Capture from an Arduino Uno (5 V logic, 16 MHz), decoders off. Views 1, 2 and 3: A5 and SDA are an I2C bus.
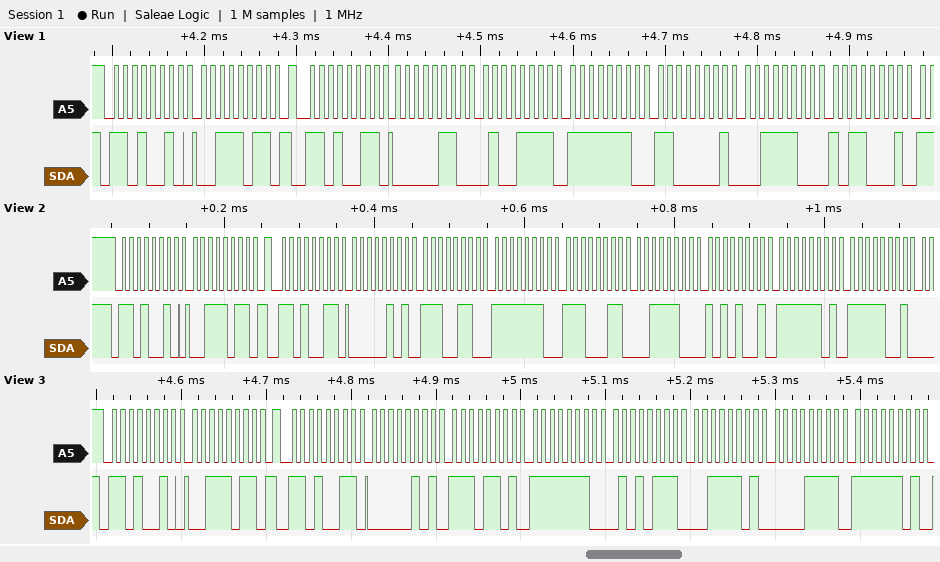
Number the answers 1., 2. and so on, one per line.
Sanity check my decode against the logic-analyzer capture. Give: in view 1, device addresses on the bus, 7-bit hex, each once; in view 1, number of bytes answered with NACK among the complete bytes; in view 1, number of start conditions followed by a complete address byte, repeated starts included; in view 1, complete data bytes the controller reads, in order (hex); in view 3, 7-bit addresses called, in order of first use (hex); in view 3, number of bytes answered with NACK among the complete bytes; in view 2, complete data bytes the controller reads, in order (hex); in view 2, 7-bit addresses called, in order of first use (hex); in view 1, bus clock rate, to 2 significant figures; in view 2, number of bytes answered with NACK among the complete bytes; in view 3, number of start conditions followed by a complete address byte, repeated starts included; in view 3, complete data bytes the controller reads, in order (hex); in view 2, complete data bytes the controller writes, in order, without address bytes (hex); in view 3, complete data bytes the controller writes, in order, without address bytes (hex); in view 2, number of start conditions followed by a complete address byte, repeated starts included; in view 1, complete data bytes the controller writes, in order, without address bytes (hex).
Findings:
1. 0x69
2. 0
3. 2
4. 06 4F FE C1 3C B1
5. 0x69
6. 0
7. 05 E6 FE E3 3C A9 FD F9
8. 0x69
9. 100 kHz
10. 0
11. 2
12. 05 ED FE 57 3D 0F FD
13. 3B
14. 3B
15. 2
16. 3B
